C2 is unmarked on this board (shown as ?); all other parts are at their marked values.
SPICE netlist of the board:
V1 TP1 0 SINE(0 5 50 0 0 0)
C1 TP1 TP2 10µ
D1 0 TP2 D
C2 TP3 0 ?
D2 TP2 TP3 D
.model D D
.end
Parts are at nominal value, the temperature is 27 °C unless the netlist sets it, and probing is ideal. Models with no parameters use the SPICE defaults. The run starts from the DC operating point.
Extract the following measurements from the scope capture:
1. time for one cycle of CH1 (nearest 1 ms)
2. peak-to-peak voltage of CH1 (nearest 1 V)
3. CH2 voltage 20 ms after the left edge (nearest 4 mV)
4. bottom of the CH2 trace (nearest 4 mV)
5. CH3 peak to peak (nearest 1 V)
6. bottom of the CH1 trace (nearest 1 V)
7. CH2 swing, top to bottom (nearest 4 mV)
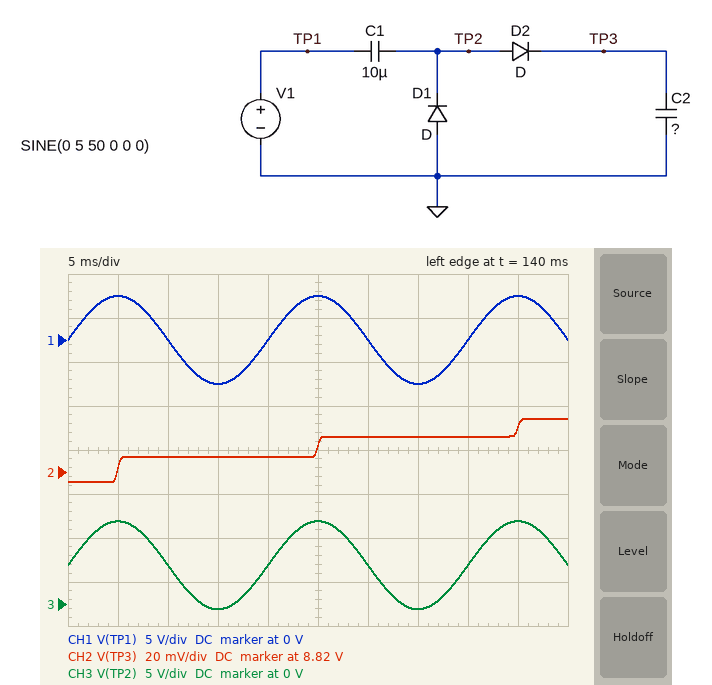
20 ms
10 V
8.828 V
8.816 V
10 V
-5 V
28 mV
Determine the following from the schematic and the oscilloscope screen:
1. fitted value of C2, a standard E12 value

2.2 µF
